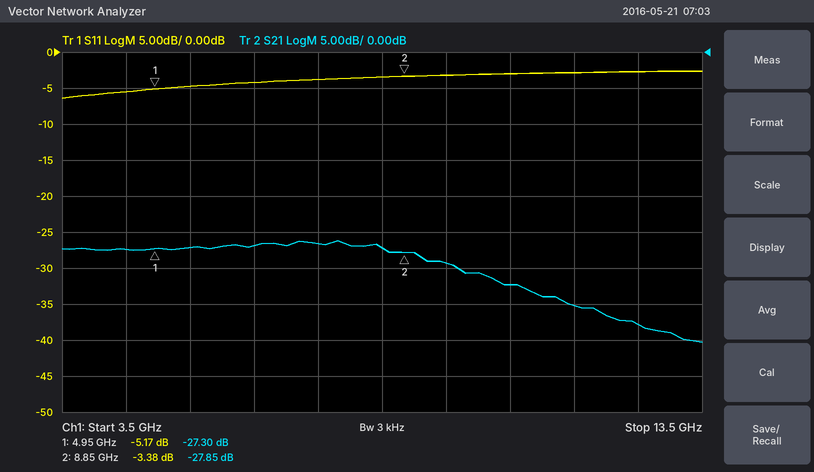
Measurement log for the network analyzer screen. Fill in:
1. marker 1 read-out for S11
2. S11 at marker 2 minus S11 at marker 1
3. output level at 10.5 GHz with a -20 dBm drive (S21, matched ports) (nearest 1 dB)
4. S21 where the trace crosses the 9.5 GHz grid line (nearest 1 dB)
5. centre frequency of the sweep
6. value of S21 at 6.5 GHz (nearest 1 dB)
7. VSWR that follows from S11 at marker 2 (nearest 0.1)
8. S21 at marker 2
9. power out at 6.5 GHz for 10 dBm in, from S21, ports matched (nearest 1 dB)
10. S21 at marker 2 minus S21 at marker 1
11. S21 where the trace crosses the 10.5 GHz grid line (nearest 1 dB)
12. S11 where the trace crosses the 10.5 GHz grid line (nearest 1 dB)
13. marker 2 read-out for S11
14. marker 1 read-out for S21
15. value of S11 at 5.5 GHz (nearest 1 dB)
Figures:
-5.17 dB
1.79 dB
-52 dBm
-29 dB
8.5 GHz
-27 dB
5.2
-27.85 dB
-17 dBm
-0.55 dB
-32 dB
-3 dB
-3.38 dB
-27.30 dB
-5 dB
